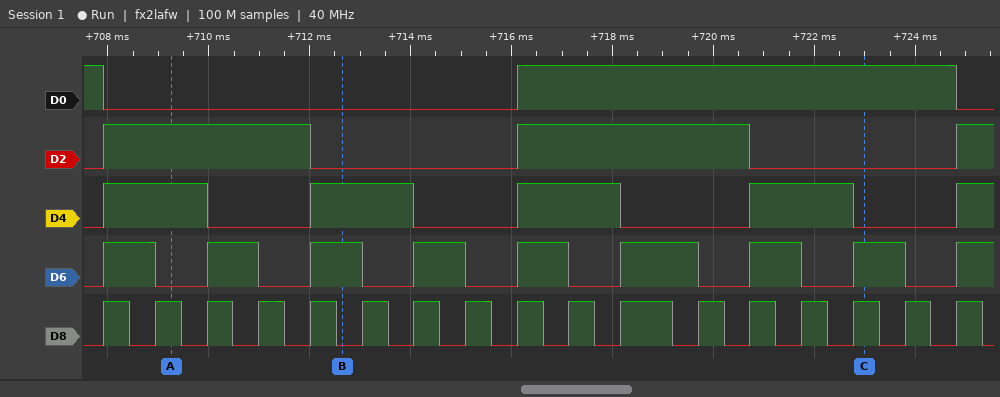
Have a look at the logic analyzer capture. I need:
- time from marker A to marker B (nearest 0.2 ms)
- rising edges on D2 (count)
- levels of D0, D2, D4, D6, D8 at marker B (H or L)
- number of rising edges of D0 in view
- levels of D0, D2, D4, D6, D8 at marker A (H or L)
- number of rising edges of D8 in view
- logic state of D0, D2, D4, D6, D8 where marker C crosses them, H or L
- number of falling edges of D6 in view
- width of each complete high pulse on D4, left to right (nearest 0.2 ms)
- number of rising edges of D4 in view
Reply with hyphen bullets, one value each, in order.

- 3.4 ms
- 3
- D0=L, D2=L, D4=H, D6=H, D8=L
- 1
- D0=L, D2=H, D4=H, D6=L, D8=H
- 17
- D0=H, D2=L, D4=L, D6=H, D8=H
- 8
- 2 ms, 2 ms, 2 ms, 2 ms
- 5
